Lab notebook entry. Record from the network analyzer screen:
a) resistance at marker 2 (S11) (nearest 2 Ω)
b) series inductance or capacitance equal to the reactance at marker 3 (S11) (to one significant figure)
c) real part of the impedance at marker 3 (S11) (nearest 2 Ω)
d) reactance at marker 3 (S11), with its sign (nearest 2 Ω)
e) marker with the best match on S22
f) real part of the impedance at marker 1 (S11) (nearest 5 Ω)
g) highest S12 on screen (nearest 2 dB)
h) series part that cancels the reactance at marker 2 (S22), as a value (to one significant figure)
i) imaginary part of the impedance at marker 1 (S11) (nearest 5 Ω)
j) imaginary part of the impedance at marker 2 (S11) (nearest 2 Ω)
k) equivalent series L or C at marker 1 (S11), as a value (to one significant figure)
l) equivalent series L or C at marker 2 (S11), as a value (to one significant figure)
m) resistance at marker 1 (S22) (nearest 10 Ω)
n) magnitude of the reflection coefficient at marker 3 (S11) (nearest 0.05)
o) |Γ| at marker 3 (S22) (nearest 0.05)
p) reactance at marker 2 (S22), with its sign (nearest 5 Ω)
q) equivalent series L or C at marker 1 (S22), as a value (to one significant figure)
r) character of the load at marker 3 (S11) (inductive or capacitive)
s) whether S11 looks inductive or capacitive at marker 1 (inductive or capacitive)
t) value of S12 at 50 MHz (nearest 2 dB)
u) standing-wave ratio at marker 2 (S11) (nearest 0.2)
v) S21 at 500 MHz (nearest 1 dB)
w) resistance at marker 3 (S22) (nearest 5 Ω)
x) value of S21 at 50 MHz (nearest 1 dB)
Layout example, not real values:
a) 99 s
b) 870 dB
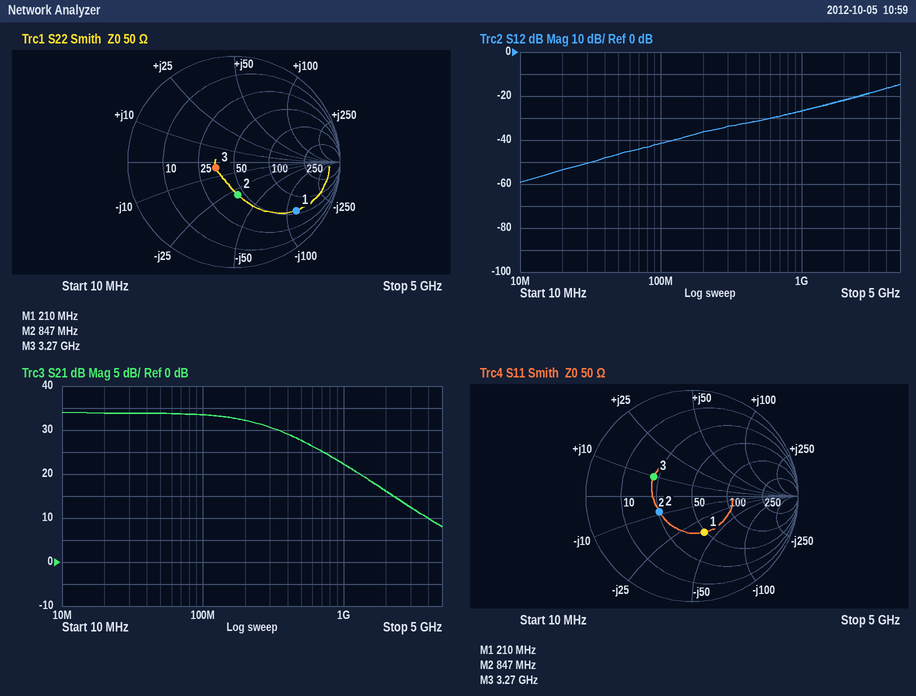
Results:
a) 26 Ω
b) 500 pH
c) 22 Ω
d) +10 Ω
e) marker 3
f) 50 Ω
g) -14 dB
h) 6 nH
i) -40 Ω
j) -8 Ω
k) 20 pF
l) 20 pF
m) 60 Ω
n) 0.40
o) 0.20
p) -30 Ω
q) 6 pF
r) inductive
s) capacitive
t) -46 dB
u) 2.0
v) 28 dB
w) 35 Ω
x) 34 dB
